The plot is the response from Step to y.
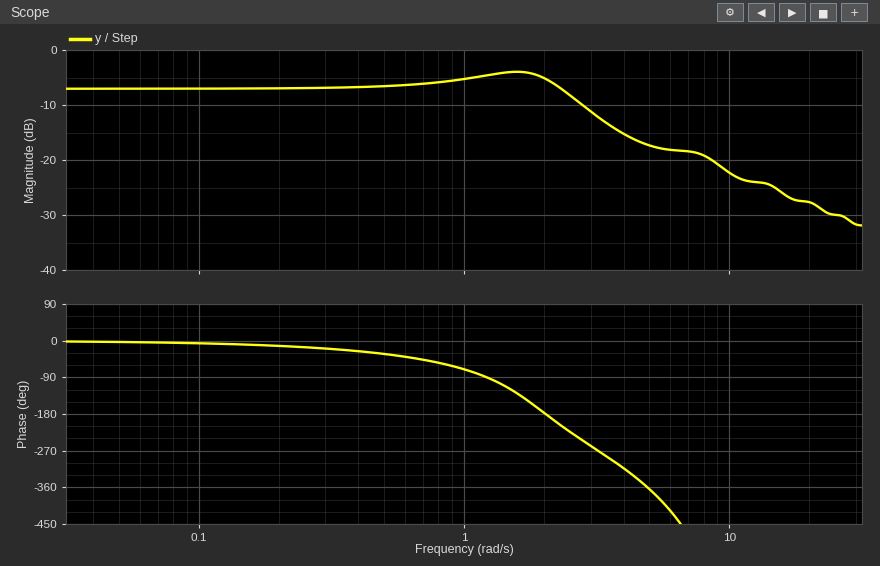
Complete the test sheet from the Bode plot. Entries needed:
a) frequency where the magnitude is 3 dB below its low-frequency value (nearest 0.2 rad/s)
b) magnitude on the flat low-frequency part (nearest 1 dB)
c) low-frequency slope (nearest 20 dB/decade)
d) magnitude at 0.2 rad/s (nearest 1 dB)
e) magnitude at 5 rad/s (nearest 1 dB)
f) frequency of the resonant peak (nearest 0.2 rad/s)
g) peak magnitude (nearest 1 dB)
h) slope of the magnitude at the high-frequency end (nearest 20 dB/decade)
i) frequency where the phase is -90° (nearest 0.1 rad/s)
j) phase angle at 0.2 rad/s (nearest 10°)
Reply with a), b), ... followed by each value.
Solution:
a) 2.8 rad/s
b) -7 dB
c) 0 dB/decade
d) -7 dB
e) -17 dB
f) 1.6 rad/s
g) -4 dB
h) -20 dB/decade
i) 1.2 rad/s
j) -10°
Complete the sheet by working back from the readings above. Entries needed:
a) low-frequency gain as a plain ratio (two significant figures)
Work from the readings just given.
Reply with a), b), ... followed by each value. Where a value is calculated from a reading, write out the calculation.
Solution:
a) 10^(-7 / 20) = 0.45
